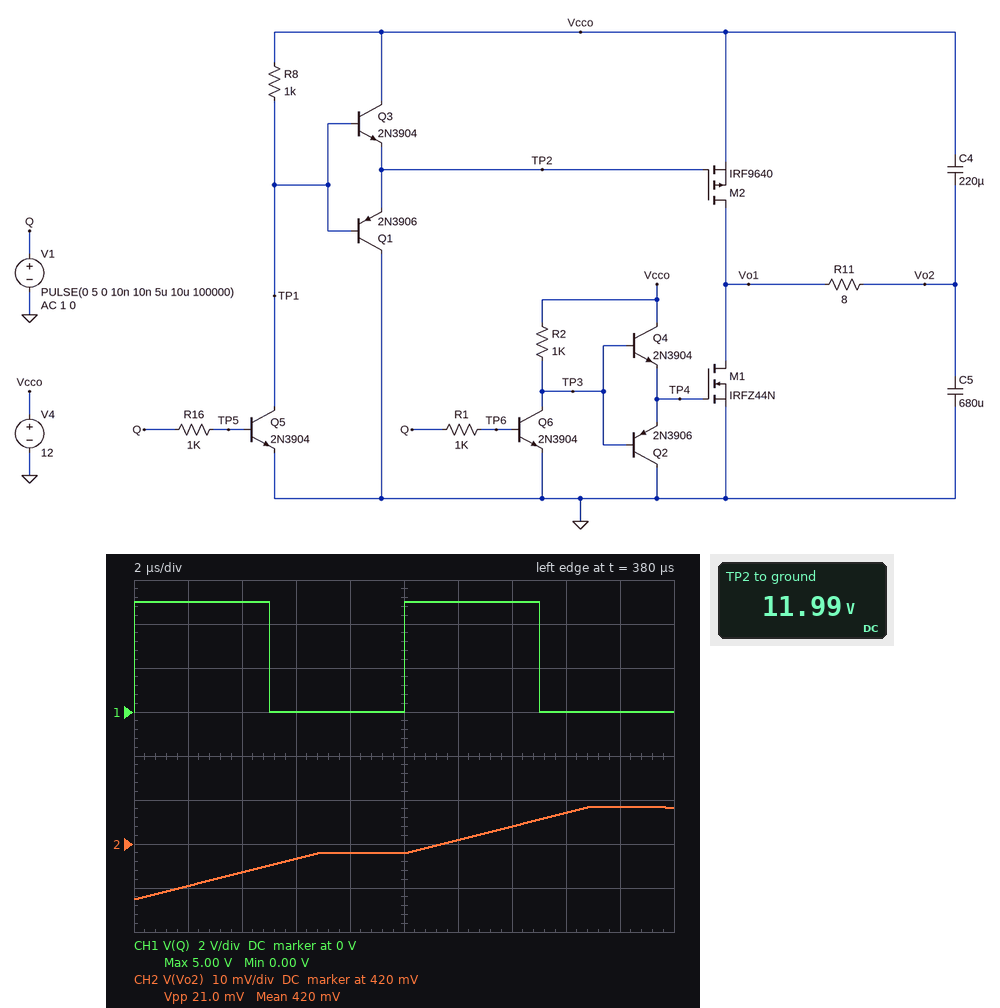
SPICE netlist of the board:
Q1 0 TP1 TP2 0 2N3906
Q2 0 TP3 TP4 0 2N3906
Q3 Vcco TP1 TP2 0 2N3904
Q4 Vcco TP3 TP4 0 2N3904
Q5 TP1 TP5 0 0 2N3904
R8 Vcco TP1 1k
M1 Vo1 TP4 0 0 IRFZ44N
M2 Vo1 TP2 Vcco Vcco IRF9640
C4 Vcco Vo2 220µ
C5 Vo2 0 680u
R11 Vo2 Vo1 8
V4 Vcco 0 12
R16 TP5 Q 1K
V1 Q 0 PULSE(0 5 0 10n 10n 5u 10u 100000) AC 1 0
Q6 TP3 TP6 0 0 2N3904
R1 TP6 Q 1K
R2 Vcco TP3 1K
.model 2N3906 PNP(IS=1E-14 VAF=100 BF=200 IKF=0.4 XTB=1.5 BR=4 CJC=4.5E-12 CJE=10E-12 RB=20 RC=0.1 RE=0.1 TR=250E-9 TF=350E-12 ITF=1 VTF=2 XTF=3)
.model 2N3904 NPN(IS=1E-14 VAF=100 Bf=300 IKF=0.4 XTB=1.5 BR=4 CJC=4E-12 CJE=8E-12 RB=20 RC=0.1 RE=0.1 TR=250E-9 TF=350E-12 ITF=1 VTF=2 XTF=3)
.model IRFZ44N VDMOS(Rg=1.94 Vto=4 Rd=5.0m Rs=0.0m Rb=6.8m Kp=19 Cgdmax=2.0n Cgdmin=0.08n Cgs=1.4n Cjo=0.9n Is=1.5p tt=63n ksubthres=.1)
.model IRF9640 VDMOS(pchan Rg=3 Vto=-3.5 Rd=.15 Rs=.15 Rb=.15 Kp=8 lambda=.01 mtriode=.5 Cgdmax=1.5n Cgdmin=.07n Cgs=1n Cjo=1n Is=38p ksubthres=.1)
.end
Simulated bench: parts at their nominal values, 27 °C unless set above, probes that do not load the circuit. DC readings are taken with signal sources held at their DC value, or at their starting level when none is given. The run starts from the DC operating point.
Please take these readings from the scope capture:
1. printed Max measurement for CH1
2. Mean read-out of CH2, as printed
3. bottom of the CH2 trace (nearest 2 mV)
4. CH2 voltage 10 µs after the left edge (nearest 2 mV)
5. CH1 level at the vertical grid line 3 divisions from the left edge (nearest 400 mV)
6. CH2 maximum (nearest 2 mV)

5.00 V
420 mV
408 mV
418 mV
0 V
428 mV
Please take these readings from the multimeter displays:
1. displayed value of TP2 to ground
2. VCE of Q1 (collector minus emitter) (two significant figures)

11.99 V
-12 V
